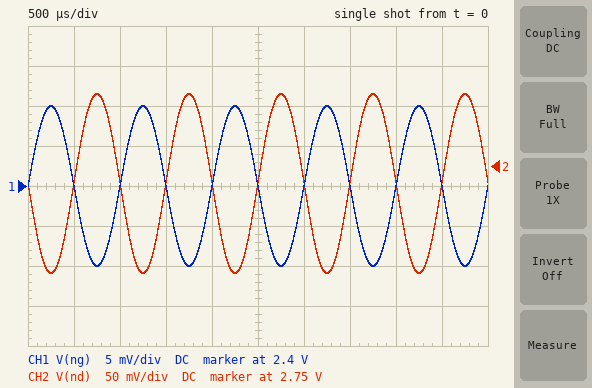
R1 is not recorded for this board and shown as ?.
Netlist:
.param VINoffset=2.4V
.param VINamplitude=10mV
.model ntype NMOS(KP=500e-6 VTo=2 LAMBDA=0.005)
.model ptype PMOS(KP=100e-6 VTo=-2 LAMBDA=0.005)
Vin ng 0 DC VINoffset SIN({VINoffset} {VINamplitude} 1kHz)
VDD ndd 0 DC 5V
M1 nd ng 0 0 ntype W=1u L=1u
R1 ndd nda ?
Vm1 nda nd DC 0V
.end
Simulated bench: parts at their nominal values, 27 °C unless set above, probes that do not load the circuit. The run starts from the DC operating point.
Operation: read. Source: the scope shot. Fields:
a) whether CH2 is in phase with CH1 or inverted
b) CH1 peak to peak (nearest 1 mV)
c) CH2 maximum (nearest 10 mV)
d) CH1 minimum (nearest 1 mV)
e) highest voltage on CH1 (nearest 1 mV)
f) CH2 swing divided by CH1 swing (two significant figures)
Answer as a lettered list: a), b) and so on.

a) inverted
b) 20 mV
c) 2.84 V
d) 2.390 V
e) 2.410 V
f) 11
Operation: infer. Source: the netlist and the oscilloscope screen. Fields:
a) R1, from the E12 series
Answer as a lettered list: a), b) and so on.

a) 56 kΩ
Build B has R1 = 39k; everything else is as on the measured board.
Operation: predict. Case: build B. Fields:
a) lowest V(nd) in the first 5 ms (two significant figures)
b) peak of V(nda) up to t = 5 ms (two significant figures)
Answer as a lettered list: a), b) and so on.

a) 3.3 V
b) 3.5 V
